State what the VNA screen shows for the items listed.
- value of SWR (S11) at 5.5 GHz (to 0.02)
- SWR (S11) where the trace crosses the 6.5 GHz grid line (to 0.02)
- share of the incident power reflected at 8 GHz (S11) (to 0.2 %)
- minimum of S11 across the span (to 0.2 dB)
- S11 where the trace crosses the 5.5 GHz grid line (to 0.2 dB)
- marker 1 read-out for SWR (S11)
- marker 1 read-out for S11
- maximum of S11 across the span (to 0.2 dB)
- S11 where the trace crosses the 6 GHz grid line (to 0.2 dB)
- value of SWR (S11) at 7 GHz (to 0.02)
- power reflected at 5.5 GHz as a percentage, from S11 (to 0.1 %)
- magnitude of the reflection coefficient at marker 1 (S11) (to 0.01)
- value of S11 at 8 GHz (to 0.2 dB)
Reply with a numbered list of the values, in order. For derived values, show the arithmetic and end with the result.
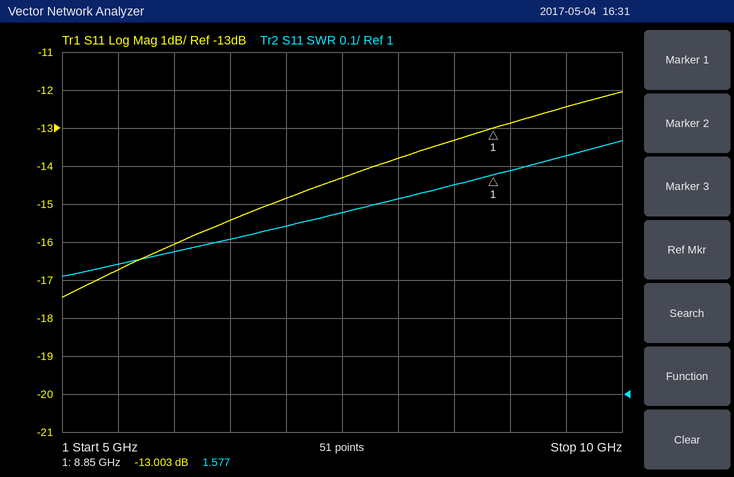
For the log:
1. 1.34
2. 1.40
3. 10^(-13.8/10) ≈ 4.2 %
4. -17.4 dB
5. -16.8 dB
6. 1.577
7. -13.003 dB
8. -12.0 dB
9. -16.0 dB
10. 1.44
11. 10^(-16.8/10) ≈ 2.1 %
12. 10^(-13.003/20) ≈ 0.22
13. -13.8 dB
